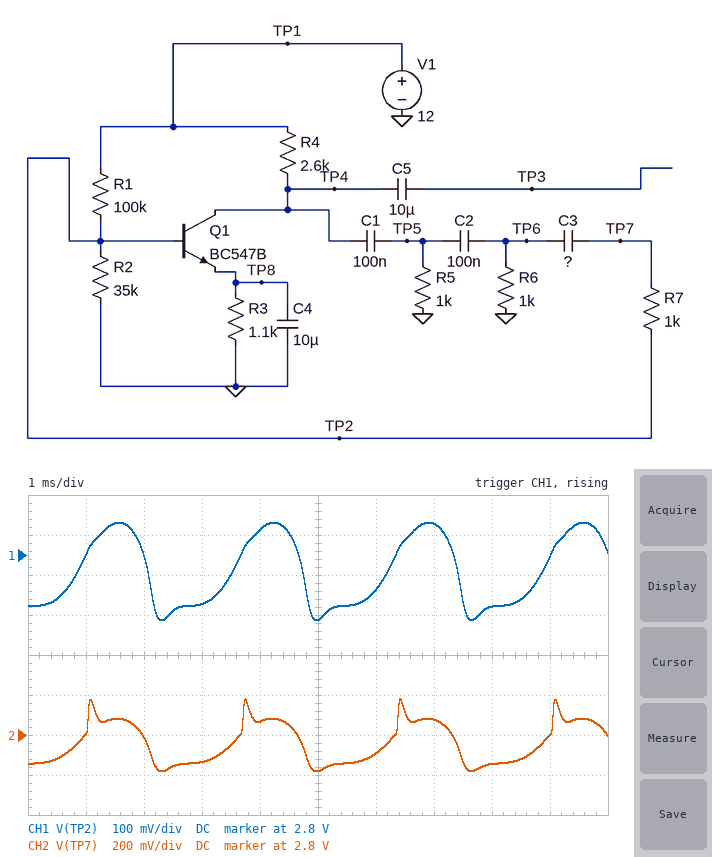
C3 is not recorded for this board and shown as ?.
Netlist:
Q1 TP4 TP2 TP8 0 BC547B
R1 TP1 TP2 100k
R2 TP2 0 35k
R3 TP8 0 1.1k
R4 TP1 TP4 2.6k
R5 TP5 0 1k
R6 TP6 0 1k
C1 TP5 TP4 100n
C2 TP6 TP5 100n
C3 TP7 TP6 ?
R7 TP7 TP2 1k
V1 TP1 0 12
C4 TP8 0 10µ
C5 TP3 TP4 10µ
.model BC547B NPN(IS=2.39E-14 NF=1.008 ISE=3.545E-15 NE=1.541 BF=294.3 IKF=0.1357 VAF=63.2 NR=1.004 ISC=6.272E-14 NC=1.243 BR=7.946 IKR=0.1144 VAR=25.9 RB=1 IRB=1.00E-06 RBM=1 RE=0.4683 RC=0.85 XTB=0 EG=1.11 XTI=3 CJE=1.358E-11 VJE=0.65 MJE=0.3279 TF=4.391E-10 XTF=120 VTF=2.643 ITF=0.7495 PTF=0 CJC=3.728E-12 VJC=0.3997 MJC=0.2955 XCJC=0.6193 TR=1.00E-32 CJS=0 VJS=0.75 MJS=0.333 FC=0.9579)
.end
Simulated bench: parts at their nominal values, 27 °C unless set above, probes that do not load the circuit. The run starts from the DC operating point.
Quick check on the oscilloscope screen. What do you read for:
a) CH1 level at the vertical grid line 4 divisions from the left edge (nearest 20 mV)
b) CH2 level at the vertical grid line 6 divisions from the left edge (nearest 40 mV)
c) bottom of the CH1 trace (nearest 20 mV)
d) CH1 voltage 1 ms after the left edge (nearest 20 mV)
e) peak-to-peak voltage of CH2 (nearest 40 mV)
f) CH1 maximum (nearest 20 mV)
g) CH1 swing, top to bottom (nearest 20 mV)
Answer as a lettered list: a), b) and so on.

a) 2.86 V
b) 2.72 V
c) 2.64 V
d) 2.80 V
e) 360 mV
f) 2.88 V
g) 240 mV
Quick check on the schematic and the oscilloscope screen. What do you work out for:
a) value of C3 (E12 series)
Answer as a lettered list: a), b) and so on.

a) 120 nF
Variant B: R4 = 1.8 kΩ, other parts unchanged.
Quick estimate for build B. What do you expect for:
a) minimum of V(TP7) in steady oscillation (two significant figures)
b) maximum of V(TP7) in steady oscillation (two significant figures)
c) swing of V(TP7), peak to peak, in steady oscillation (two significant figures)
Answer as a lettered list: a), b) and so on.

a) 2.8 V
b) 3.1 V
c) 330 mV
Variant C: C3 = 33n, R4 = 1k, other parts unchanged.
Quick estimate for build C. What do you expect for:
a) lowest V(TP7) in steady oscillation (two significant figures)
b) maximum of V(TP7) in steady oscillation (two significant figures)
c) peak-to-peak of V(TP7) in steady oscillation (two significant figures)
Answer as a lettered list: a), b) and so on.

a) 2.8 V
b) 3.1 V
c) 280 mV
